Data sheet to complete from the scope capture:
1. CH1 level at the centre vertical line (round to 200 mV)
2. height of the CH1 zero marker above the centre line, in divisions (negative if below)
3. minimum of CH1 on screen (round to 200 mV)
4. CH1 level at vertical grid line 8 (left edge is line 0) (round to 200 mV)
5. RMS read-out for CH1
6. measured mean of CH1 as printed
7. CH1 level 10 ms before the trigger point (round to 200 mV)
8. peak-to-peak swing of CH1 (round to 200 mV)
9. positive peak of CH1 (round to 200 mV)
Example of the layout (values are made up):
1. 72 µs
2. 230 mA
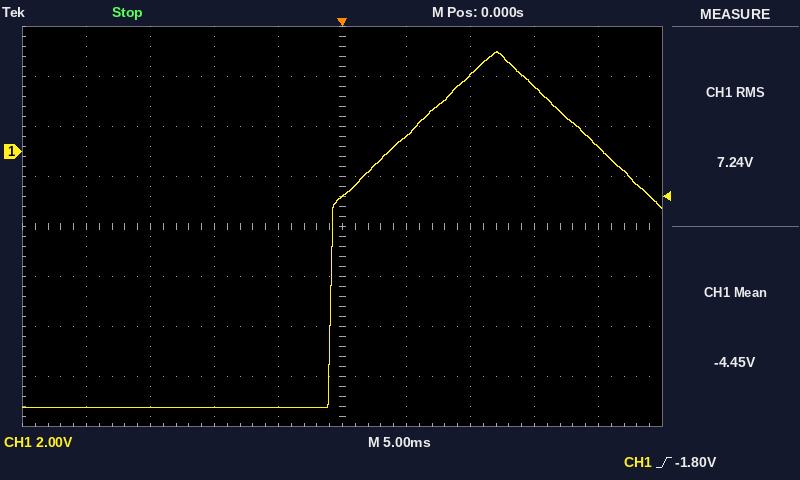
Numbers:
1. -1.8 V
2. +1.5 div
3. -10.2 V
4. 2.6 V
5. 7.24 V
6. -4.45 V
7. -10.2 V
8. 14.2 V
9. 4.0 V
